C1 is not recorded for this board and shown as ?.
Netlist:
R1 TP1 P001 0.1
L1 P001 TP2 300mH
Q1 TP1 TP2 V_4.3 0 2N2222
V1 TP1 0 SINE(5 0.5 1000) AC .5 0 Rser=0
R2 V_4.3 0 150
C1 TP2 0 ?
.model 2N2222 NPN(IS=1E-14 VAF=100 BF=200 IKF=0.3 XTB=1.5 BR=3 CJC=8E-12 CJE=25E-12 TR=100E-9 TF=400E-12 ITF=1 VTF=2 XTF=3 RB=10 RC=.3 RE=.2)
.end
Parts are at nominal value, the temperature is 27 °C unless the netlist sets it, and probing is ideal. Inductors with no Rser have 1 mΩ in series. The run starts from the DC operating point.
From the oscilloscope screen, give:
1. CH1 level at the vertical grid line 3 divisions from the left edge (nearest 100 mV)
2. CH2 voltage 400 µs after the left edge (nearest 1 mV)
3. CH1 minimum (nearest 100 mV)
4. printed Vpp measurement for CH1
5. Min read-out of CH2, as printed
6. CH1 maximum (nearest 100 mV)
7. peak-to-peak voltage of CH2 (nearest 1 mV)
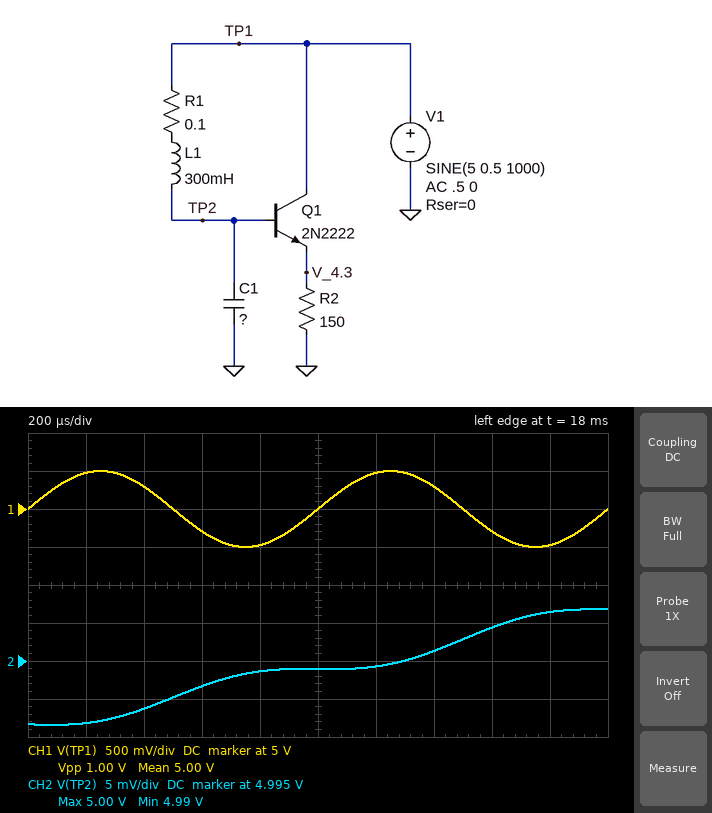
4.7 V
4.989 V
4.5 V
1.00 V
4.99 V
5.5 V
15 mV
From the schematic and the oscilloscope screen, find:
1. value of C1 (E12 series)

33 µF
